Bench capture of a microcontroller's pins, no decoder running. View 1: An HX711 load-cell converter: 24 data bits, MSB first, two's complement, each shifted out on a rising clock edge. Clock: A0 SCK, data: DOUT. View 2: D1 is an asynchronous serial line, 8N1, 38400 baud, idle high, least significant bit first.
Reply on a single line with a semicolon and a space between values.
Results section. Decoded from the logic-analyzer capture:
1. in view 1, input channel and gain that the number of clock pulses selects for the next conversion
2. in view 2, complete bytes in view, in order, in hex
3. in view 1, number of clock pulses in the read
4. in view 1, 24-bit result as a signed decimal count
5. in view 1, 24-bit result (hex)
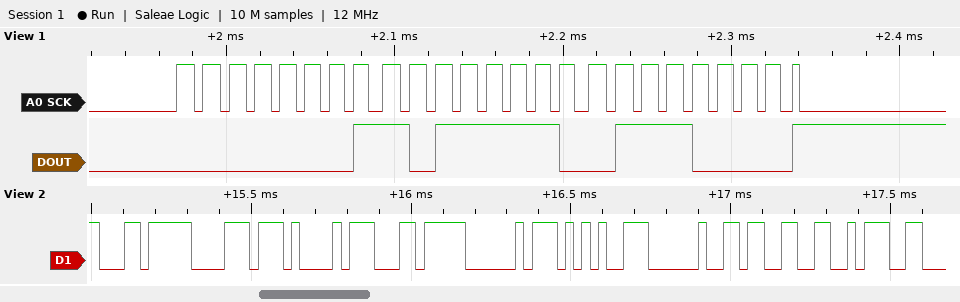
channel A, gain 128; EC B8 A1 EC A0 95 20 33 3A; 25; 114288; 0x01BE70
